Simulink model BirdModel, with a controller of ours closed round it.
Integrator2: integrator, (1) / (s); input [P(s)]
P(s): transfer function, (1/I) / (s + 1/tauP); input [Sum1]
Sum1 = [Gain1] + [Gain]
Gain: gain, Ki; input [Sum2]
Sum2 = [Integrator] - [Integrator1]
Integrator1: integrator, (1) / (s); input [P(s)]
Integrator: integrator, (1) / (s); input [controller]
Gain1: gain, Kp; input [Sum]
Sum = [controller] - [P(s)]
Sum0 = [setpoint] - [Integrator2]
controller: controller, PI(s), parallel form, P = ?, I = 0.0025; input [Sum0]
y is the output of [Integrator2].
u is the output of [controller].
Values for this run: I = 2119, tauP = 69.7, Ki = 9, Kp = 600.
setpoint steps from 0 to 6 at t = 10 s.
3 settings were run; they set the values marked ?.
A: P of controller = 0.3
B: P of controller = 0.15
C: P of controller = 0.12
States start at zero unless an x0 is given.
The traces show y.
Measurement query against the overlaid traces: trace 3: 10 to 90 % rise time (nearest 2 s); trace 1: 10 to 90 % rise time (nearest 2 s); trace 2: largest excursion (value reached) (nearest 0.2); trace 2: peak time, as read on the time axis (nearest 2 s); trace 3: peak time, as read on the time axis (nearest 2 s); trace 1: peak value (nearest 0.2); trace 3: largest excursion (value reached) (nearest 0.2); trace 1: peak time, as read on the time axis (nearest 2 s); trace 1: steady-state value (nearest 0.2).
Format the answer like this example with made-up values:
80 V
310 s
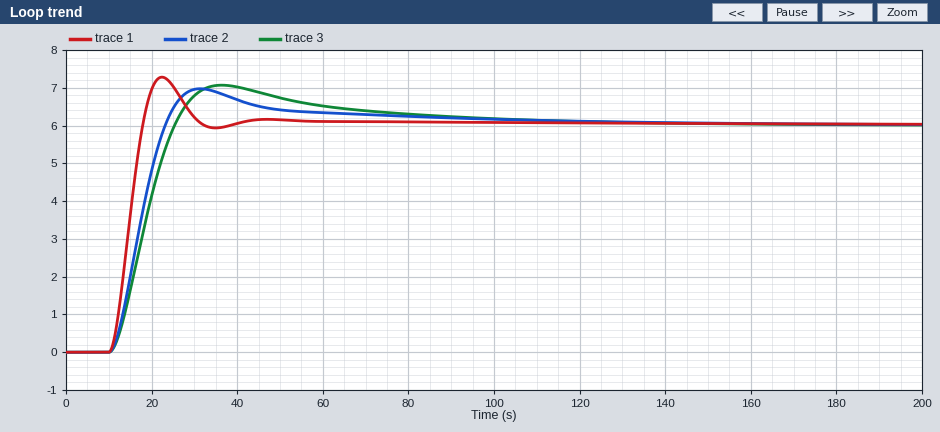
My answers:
10 s
6 s
7.0
32 s
36 s
7.2
7.0
22 s
6.0
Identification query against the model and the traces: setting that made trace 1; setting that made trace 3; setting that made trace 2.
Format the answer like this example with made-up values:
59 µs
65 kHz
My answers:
A
C
B
